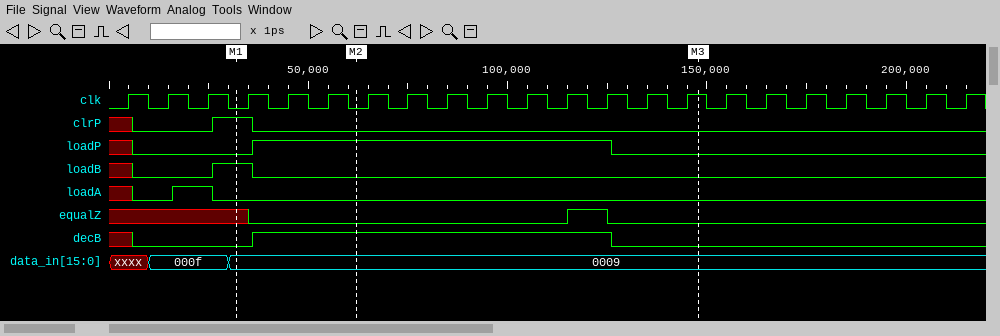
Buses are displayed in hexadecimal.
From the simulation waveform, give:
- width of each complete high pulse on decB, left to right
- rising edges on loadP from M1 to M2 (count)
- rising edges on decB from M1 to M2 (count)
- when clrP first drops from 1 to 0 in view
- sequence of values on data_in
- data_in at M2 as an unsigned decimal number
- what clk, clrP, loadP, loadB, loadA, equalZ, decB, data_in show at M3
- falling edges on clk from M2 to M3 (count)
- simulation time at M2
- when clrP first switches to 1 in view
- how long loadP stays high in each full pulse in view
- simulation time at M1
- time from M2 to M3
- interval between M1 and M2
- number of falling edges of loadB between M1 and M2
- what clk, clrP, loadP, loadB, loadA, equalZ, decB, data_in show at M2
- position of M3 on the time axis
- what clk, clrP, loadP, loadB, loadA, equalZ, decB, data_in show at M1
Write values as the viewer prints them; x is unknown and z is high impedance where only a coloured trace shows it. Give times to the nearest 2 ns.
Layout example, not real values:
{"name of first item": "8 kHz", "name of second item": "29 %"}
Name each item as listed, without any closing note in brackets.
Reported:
{"width of each complete high pulse on decB, left to right": "90 ns", "rising edges on loadP from M1 to M2": "1", "rising edges on decB from M1 to M2": "1", "when clrP first drops from 1 to 0 in view": "36 ns", "sequence of values on data_in": "xxxx, 000f, 0009", "data_in at M2 as an unsigned decimal number": "9", "what clk, clrP, loadP, loadB, loadA, equalZ, decB, data_in show at M3": "clk=1, clrP=0, loadP=0, loadB=0, loadA=0, equalZ=0, decB=0, data_in=0009", "falling edges on clk from M2 to M3": "8", "simulation time at M2": "62 ns", "when clrP first switches to 1 in view": "26 ns", "how long loadP stays high in each full pulse in view": "90 ns", "simulation time at M1": "32 ns", "time from M2 to M3": "86 ns", "interval between M1 and M2": "30 ns", "number of falling edges of loadB between M1 and M2": "1", "what clk, clrP, loadP, loadB, loadA, equalZ, decB, data_in show at M2": "clk=0, clrP=0, loadP=1, loadB=0, loadA=0, equalZ=0, decB=1, data_in=0009", "position of M3 on the time axis": "148 ns", "what clk, clrP, loadP, loadB, loadA, equalZ, decB, data_in show at M1": "clk=0, clrP=1, loadP=0, loadB=1, loadA=0, equalZ=x, decB=0, data_in=0009"}
